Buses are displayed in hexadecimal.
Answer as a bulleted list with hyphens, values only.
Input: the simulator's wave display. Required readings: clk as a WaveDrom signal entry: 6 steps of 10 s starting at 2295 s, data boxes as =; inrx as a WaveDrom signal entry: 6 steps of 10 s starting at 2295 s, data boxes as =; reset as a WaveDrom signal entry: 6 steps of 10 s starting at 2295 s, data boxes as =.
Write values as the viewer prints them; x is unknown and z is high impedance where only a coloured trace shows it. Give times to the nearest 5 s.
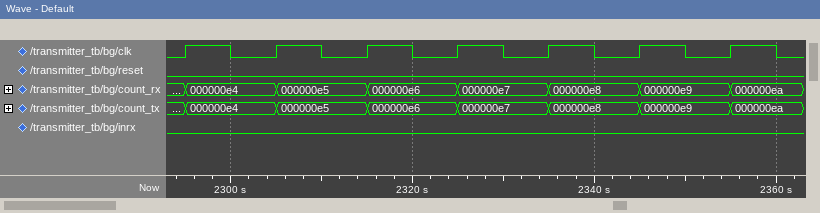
- {name: 'clk', wave: 'p.....'}
- {name: 'inrx', wave: '0.....'}
- {name: 'reset', wave: '0.....'}
